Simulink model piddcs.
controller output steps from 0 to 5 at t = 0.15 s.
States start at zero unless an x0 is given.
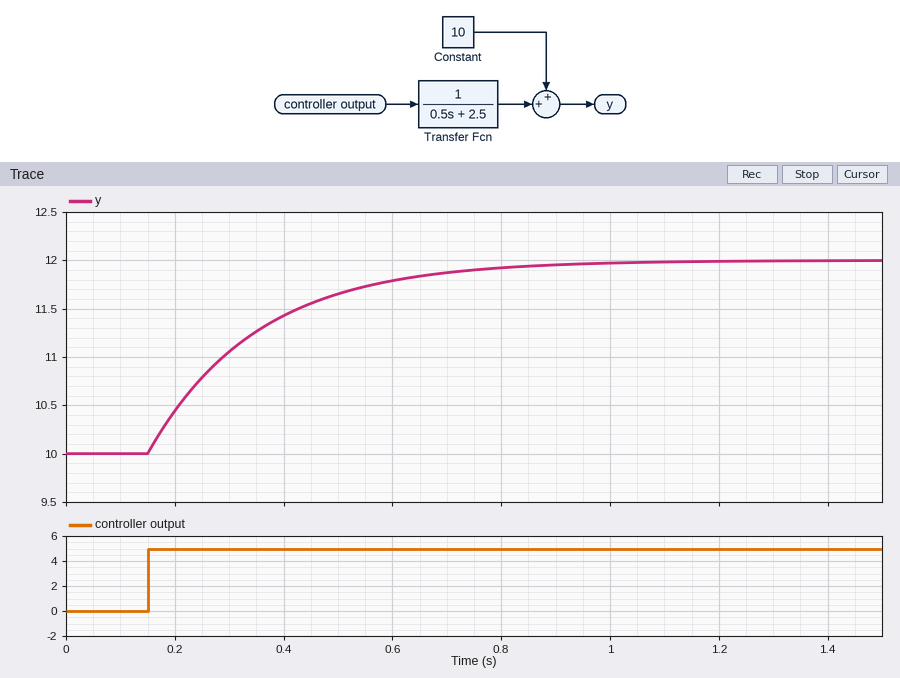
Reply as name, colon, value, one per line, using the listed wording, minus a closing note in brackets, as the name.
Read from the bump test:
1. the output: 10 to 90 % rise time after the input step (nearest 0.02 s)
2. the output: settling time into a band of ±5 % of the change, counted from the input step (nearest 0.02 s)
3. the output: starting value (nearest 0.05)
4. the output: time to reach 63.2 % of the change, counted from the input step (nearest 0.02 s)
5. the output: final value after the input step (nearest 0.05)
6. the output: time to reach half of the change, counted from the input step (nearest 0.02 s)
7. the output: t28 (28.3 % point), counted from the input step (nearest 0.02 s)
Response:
the output: 10 to 90 % rise time after the input step: 0.44 s
the output: settling time into a band of ±5 % of the change, counted from the input step: 0.60 s
the output: starting value: 10.00
the output: time to reach 63.2 % of the change, counted from the input step: 0.20 s
the output: final value after the input step: 12.00
the output: time to reach half of the change, counted from the input step: 0.14 s
the output: t28 (28.3 % point), counted from the input step: 0.06 s
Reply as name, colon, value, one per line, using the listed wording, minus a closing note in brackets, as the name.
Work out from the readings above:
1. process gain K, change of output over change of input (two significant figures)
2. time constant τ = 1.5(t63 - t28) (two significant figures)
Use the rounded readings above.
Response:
process gain K, change of output over change of input: 0.40
time constant τ = 1.5(t63 - t28): 0.21 s
